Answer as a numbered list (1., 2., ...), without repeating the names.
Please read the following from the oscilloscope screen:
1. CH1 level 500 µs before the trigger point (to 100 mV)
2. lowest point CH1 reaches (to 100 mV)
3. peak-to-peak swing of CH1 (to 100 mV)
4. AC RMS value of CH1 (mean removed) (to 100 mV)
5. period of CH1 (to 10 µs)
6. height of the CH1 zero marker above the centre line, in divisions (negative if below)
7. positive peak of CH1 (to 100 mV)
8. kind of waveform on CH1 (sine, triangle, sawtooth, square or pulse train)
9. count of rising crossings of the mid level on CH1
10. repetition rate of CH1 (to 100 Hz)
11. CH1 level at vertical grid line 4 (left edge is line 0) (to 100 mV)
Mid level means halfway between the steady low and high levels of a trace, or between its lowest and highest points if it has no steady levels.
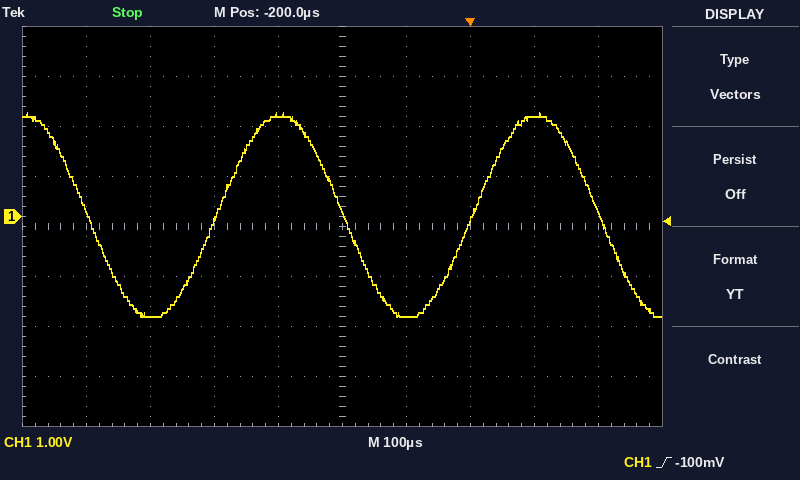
1. -2.0 V
2. -2.0 V
3. 4.1 V
4. 1.4 V
5. 400 µs
6. +0.2 div
7. 2.1 V
8. sine
9. 2
10. 2.5 kHz
11. 2.0 V
